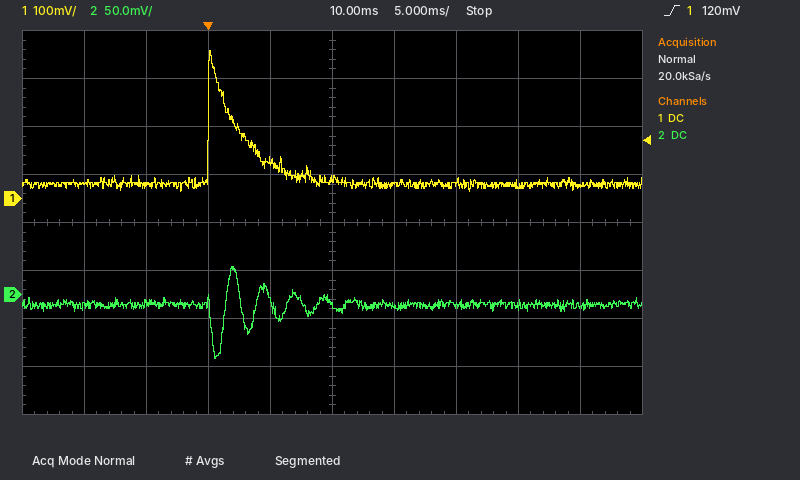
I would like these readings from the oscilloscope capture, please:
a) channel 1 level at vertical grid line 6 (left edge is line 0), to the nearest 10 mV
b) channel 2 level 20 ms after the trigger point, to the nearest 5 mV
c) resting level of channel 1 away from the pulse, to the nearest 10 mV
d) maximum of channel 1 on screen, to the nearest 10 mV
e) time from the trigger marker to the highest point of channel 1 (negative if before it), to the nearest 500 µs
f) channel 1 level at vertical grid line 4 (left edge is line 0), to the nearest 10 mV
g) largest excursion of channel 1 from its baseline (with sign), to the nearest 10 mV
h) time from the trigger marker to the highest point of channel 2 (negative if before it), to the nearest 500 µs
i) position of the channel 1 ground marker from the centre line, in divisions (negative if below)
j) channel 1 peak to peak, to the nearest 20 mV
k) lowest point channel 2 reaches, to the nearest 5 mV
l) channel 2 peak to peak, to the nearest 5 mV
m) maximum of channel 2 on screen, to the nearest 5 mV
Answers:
30 mV
-10 mV
30 mV
310 mV
0.0 ms
80 mV
+280 mV
+2.0 ms
+0.5 div
300 mV
-65 mV
95 mV
30 mV
